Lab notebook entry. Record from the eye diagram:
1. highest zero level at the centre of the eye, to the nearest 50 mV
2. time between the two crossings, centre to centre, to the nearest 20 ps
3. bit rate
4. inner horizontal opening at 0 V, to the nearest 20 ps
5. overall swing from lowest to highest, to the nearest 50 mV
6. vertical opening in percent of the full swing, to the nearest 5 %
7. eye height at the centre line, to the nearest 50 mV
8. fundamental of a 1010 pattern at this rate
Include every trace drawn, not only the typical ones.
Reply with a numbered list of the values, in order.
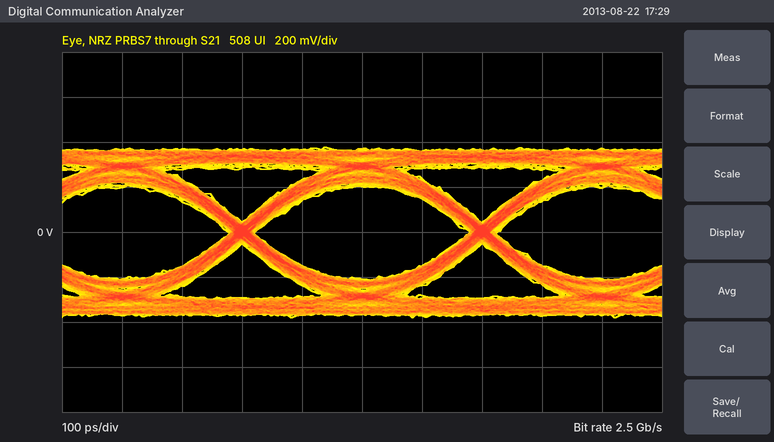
1. -200 mV
2. 400 ps
3. 2.5 Gb/s
4. 360 ps
5. 750 mV
6. 55 %
7. 400 mV
8. 1.25 GHz
